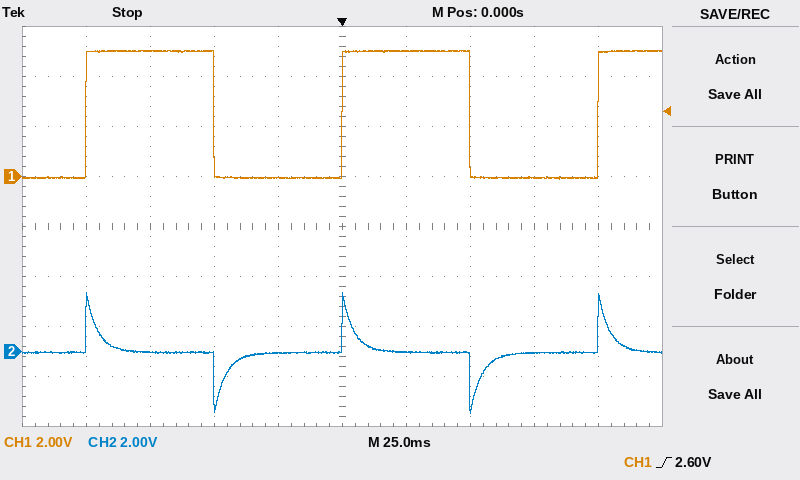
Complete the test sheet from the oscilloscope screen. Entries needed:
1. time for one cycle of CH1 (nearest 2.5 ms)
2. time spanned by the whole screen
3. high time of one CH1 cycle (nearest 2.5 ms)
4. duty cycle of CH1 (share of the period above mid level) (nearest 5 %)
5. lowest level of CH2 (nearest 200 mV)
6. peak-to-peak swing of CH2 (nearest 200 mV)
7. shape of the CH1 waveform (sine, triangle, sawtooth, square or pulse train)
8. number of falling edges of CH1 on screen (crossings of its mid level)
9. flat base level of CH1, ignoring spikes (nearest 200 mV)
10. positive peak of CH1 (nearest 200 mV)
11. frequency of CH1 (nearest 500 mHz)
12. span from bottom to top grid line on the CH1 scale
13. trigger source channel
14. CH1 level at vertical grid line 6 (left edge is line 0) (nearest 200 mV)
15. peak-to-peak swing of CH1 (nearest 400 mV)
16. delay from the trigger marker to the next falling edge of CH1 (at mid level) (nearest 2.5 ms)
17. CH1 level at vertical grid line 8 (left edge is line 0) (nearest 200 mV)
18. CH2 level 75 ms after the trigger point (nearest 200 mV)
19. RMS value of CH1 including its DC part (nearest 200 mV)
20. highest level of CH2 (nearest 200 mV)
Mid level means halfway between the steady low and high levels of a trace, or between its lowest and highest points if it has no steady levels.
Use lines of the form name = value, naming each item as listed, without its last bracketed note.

time for one cycle of CH1 = 100.0 ms
time spanned by the whole screen = 250 ms
high time of one CH1 cycle = 50.0 ms
duty cycle of CH1 (share of the period above mid level) = 50 %
lowest level of CH2 = -2.4 V
peak-to-peak swing of CH2 = 4.8 V
shape of the CH1 waveform = square
number of falling edges of CH1 on screen = 2
flat base level of CH1, ignoring spikes = 0.0 V
positive peak of CH1 = 5.0 V
frequency of CH1 = 10.0 Hz
span from bottom to top grid line on the CH1 scale = 16 V
trigger source channel = CH1
CH1 level at vertical grid line 6 (left edge is line 0) = 5.0 V
peak-to-peak swing of CH1 = 5.2 V
delay from the trigger marker to the next falling edge of CH1 (at mid level) = 50.0 ms
CH1 level at vertical grid line 8 (left edge is line 0) = 0.0 V
CH2 level 75 ms after the trigger point = 0.0 V
RMS value of CH1 including its DC part = 3.6 V
highest level of CH2 = 2.4 V
